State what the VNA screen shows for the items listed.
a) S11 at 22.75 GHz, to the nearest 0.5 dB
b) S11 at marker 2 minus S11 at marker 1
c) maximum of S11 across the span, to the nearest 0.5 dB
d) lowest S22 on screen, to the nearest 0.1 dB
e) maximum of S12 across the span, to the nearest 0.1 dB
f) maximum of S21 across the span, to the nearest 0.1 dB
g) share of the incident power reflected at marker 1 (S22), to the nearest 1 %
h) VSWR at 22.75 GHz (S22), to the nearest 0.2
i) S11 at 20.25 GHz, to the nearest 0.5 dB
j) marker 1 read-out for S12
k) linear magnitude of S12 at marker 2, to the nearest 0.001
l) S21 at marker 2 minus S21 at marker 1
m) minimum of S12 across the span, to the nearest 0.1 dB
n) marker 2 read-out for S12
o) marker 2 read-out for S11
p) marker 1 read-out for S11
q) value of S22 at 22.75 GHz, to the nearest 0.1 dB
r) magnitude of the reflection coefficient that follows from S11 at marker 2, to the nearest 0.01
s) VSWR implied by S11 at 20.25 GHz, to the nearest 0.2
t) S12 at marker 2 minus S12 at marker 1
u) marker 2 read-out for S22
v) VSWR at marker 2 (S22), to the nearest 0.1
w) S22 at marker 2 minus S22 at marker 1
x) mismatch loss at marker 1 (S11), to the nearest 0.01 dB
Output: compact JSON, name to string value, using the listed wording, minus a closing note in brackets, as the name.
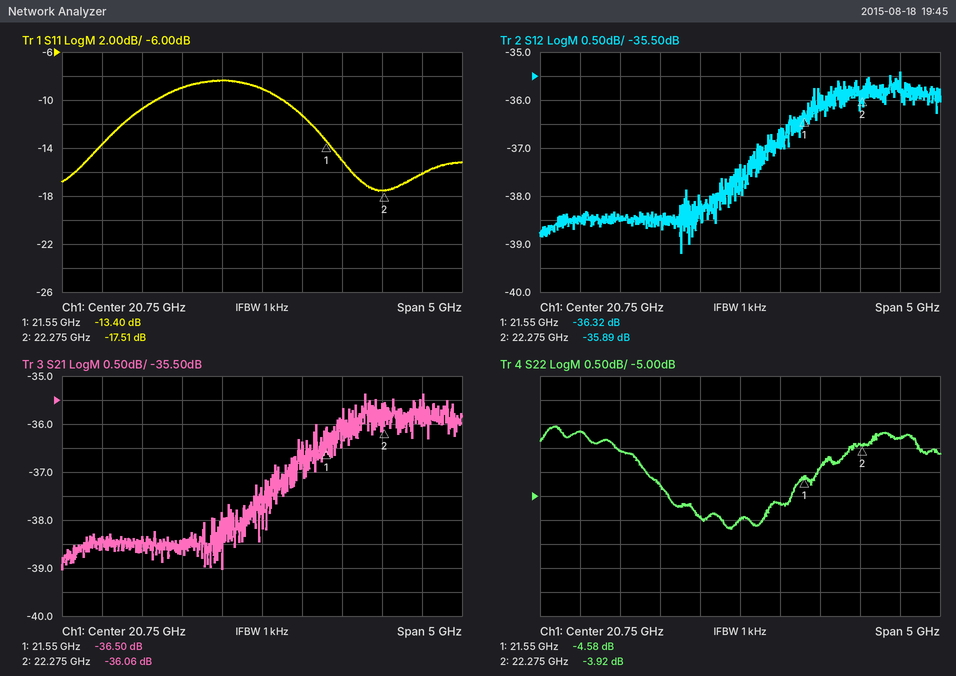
{"S11 at 22.75 GHz, to the nearest 0.5 dB": "-16.0 dB", "S11 at marker 2 minus S11 at marker 1": "-4.11 dB", "maximum of S11 across the span, to the nearest 0.5 dB": "-8.5 dB", "lowest S22 on screen, to the nearest 0.1 dB": "-5.7 dB", "maximum of S12 across the span, to the nearest 0.1 dB": "-35.4 dB", "maximum of S21 across the span, to the nearest 0.1 dB": "-35.4 dB", "share of the incident power reflected at marker 1 (S22), to the nearest 1 %": "35 %", "VSWR at 22.75 GHz (S22), to the nearest 0.2": "4.6", "S11 at 20.25 GHz, to the nearest 0.5 dB": "-8.5 dB", "marker 1 read-out for S12": "-36.32 dB", "linear magnitude of S12 at marker 2, to the nearest 0.001": "0.016", "S21 at marker 2 minus S21 at marker 1": "0.44 dB", "minimum of S12 across the span, to the nearest 0.1 dB": "-39.2 dB", "marker 2 read-out for S12": "-35.89 dB", "marker 2 read-out for S11": "-17.51 dB", "marker 1 read-out for S11": "-13.40 dB", "value of S22 at 22.75 GHz, to the nearest 0.1 dB": "-3.8 dB", "magnitude of the reflection coefficient that follows from S11 at marker 2, to the nearest 0.01": "0.13", "VSWR implied by S11 at 20.25 GHz, to the nearest 0.2": "2.2", "S12 at marker 2 minus S12 at marker 1": "0.43 dB", "marker 2 read-out for S22": "-3.92 dB", "VSWR at marker 2 (S22), to the nearest 0.1": "4.5", "S22 at marker 2 minus S22 at marker 1": "0.66 dB", "mismatch loss at marker 1 (S11), to the nearest 0.01 dB": "0.20 dB"}
